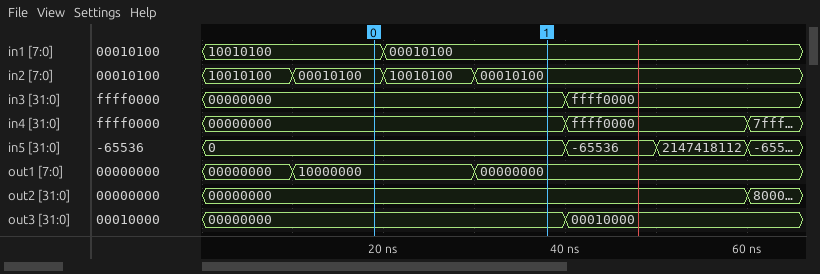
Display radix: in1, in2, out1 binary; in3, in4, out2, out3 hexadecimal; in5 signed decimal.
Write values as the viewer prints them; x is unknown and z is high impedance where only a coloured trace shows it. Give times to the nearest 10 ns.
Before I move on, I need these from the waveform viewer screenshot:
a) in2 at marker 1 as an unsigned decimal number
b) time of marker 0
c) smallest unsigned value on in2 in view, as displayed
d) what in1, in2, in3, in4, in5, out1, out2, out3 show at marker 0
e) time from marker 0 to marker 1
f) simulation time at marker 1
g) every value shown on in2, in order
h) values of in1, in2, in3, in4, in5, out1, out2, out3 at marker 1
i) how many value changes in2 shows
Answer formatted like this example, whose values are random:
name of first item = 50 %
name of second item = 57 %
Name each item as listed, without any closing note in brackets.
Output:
in2 at marker 1 as an unsigned decimal number = 20
time of marker 0 = 20 ns
smallest unsigned value on in2 in view, as displayed = 00010100
what in1, in2, in3, in4, in5, out1, out2, out3 show at marker 0 = in1=10010100, in2=00010100, in3=00000000, in4=00000000, in5=0, out1=10000000, out2=00000000, out3=00000000
time from marker 0 to marker 1 = 20 ns
simulation time at marker 1 = 40 ns
every value shown on in2, in order = 10010100, 00010100, 10010100, 00010100
values of in1, in2, in3, in4, in5, out1, out2, out3 at marker 1 = in1=00010100, in2=00010100, in3=00000000, in4=00000000, in5=0, out1=00000000, out2=00000000, out3=00000000
how many value changes in2 shows = 3
